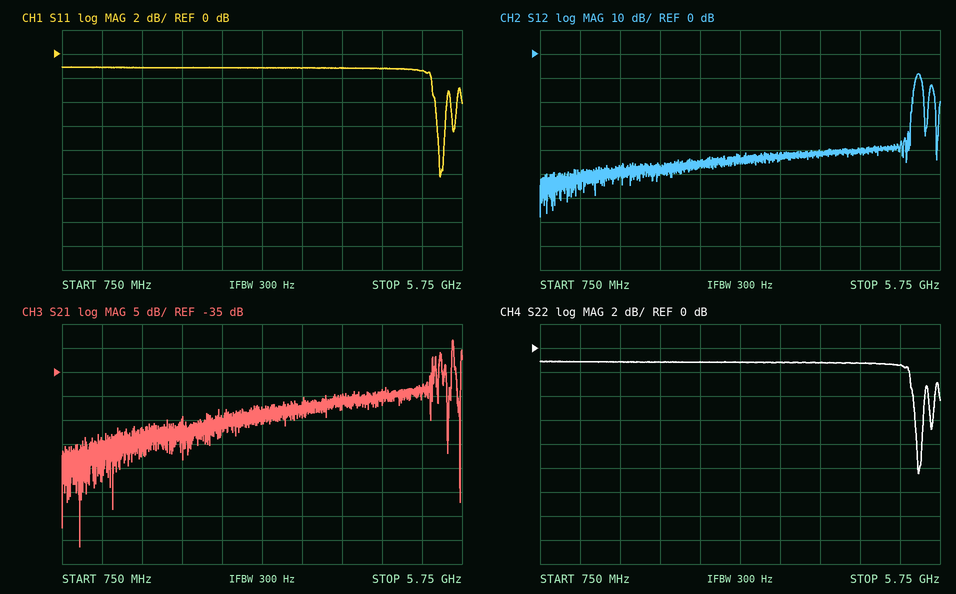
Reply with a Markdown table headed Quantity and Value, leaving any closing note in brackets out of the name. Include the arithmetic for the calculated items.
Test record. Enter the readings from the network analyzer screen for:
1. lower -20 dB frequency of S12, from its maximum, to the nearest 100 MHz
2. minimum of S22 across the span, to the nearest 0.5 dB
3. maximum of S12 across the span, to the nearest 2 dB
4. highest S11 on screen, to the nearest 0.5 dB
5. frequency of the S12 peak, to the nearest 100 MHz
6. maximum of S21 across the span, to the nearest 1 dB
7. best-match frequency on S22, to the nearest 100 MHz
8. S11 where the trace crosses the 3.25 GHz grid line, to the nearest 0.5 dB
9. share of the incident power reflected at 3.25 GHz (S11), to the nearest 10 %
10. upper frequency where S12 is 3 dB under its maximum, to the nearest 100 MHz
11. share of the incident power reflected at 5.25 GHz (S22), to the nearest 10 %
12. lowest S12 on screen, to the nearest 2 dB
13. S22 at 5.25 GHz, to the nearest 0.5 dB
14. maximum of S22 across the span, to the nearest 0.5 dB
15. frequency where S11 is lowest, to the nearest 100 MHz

| Quantity | Value |
|---|---|
| lower -20 dB frequency of S12, from its maximum, to the nearest 100 MHz | 5.4 GHz |
| minimum of S22 across the span, to the nearest 0.5 dB | -10.5 dB |
| maximum of S12 across the span, to the nearest 2 dB | -8 dB |
| highest S11 on screen, to the nearest 0.5 dB | -1.0 dB |
| frequency of the S12 peak, to the nearest 100 MHz | 5.5 GHz |
| maximum of S21 across the span, to the nearest 1 dB | -28 dB |
| best-match frequency on S22, to the nearest 100 MHz | 5.5 GHz |
| S11 where the trace crosses the 3.25 GHz grid line, to the nearest 0.5 dB | -1.0 dB |
| share of the incident power reflected at 3.25 GHz (S11), to the nearest 10 % | 10^(-1/10) ≈ 79.4 %, so 80 % to the nearest 10 % |
| upper frequency where S12 is 3 dB under its maximum, to the nearest 100 MHz | 5.5 GHz |
| share of the incident power reflected at 5.25 GHz (S22), to the nearest 10 % | 10^(-1.5/10) ≈ 70.8 %, so 70 % to the nearest 10 % |
| lowest S12 on screen, to the nearest 2 dB | -68 dB |
| S22 at 5.25 GHz, to the nearest 0.5 dB | -1.5 dB |
| maximum of S22 across the span, to the nearest 0.5 dB | -1.0 dB |
| frequency where S11 is lowest, to the nearest 100 MHz | 5.5 GHz |
